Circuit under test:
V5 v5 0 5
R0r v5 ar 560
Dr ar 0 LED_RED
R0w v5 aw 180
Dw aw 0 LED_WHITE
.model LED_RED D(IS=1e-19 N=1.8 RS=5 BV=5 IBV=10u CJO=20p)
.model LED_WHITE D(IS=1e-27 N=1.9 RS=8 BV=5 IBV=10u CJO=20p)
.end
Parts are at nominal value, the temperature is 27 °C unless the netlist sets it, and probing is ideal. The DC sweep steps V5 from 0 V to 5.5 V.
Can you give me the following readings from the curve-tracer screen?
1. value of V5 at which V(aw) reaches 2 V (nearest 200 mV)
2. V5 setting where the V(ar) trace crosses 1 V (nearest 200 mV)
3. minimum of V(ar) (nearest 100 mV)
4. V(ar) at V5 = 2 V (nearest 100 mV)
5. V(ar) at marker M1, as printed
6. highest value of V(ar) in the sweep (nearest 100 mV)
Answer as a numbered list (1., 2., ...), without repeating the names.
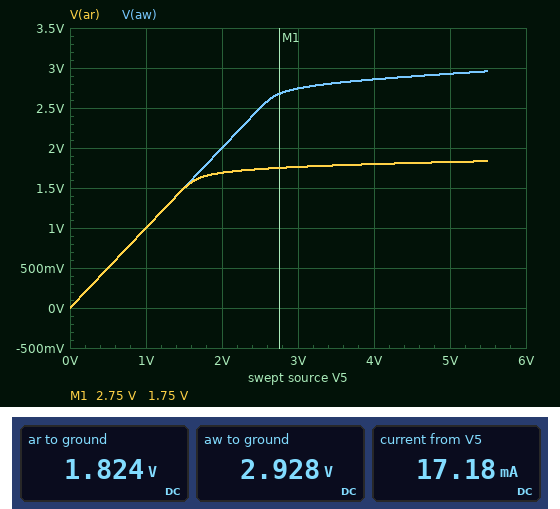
1. 2.0 V
2. 1.0 V
3. 0 V
4. 1.7 V
5. 1.75 V
6. 1.8 V
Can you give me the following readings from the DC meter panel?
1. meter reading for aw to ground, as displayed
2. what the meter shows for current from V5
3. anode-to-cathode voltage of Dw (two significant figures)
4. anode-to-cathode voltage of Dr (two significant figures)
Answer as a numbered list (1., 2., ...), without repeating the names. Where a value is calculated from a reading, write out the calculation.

1. 2.928 V
2. 17.18 mA
3. 2.928 V = 2.9 V
4. 1.824 V = 1.8 V
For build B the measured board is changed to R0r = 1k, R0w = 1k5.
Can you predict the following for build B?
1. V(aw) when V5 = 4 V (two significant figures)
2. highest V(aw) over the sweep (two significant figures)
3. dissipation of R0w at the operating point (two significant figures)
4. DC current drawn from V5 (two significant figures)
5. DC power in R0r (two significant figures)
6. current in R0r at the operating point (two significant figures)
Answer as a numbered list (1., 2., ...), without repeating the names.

1. 2.7 V
2. 2.8 V
3. 3.4 mW
4. 4.7 mA
5. 10 mW
6. 3.2 mA
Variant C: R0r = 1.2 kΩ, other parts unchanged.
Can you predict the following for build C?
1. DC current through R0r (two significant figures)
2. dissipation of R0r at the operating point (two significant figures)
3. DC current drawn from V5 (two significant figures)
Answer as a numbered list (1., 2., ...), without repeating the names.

1. 2.7 mA
2. 8.7 mW
3. 14 mA
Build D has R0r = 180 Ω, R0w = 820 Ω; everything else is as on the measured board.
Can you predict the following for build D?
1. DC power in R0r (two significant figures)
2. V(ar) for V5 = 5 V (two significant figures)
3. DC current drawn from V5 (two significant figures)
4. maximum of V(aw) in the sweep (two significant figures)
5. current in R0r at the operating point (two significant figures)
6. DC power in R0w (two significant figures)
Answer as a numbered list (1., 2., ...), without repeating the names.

1. 52 mW
2. 1.9 V
3. 20 mA
4. 2.8 V
5. 17 mA
6. 6.0 mW
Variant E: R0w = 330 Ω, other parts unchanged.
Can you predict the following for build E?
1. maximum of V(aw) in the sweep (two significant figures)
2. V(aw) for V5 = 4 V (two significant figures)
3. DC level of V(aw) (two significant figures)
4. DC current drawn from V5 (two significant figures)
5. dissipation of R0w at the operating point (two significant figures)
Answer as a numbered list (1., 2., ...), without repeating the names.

1. 2.9 V
2. 2.8 V
3. 2.9 V
4. 12 mA
5. 14 mW
